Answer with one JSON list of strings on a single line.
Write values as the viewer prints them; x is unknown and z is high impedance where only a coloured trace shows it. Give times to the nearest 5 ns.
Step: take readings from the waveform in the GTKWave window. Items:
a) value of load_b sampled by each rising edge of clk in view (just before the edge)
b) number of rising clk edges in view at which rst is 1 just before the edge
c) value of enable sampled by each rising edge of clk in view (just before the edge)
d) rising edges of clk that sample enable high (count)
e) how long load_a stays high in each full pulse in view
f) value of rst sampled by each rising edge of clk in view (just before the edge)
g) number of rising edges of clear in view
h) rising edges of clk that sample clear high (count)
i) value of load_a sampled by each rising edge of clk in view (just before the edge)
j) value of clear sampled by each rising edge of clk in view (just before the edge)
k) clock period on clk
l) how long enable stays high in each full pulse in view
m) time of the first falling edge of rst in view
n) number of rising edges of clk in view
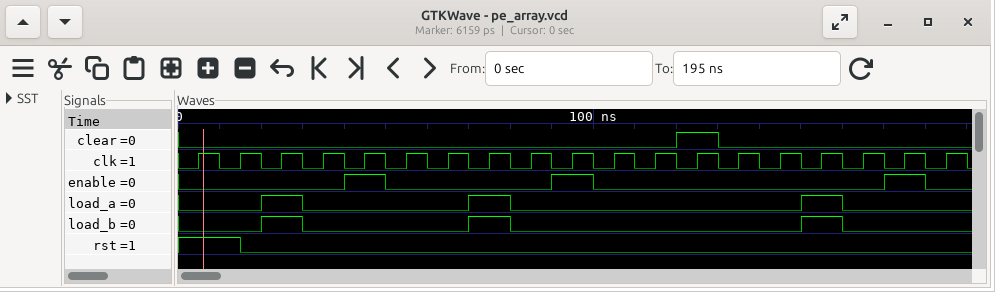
["0 0 1 0 0 0 0 1 0 0 0 0 0 0 0 1 0 0 0", "2", "0 0 0 0 1 0 0 0 0 1 0 0 0 0 0 0 0 1 0", "3", "10 ns, 10 ns, 10 ns", "1 1 0 0 0 0 0 0 0 0 0 0 0 0 0 0 0 0 0", "1", "1", "0 0 1 0 0 0 0 1 0 0 0 0 0 0 0 1 0 0 0", "0 0 0 0 0 0 0 0 0 0 0 0 1 0 0 0 0 0 0", "10 ns", "10 ns, 10 ns, 10 ns", "15 ns", "19"]
